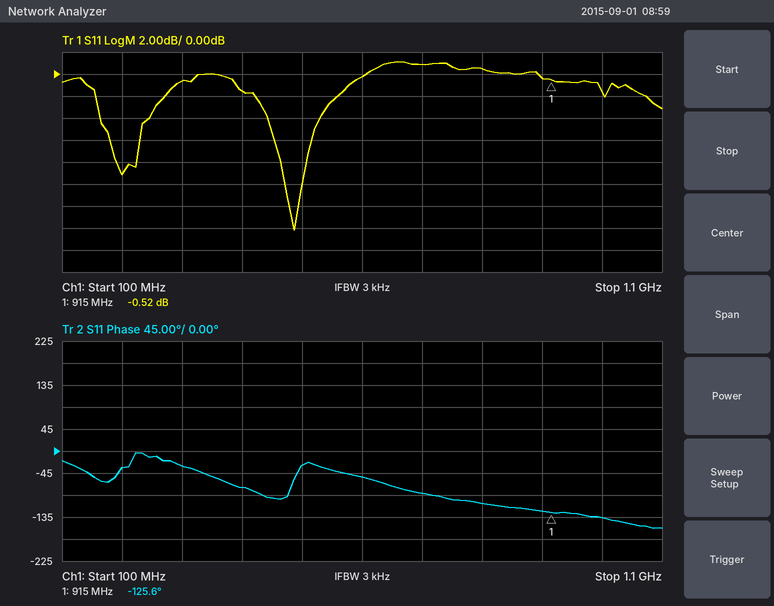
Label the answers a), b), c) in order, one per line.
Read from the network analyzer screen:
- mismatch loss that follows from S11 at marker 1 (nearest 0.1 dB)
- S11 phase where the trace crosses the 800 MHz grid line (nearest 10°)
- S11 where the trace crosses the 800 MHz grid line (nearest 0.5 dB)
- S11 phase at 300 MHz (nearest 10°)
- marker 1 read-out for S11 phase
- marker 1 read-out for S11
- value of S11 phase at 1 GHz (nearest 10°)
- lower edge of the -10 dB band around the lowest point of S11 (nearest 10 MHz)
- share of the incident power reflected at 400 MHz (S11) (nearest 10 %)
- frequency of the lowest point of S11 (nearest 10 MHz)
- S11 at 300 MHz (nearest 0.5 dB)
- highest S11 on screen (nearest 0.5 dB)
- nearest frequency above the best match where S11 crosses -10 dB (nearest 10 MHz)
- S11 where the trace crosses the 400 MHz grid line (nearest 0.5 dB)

a) 9.5 dB
b) -110°
c) 0.5 dB
d) -30°
e) -125.6°
f) -0.52 dB
g) -140°
h) 470 MHz
i) 70 %
j) 490 MHz
k) -0.5 dB
l) 1.0 dB
m) 500 MHz
n) -1.5 dB
